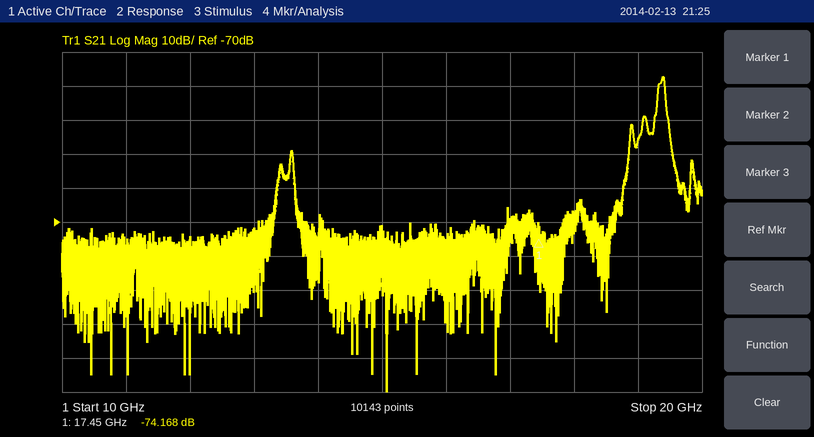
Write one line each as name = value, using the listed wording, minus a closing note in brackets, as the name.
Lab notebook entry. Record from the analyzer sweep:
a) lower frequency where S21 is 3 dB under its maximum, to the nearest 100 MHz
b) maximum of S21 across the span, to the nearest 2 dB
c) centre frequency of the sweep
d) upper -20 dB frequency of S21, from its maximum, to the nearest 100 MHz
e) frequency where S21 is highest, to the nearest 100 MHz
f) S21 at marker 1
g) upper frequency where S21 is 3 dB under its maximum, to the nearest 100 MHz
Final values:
lower frequency where S21 is 3 dB under its maximum, to the nearest 100 MHz = 19.3 GHz
maximum of S21 across the span, to the nearest 2 dB = -28 dB
centre frequency of the sweep = 15 GHz
upper -20 dB frequency of S21, from its maximum, to the nearest 100 MHz = 19.5 GHz
frequency where S21 is highest, to the nearest 100 MHz = 19.4 GHz
S21 at marker 1 = -74.168 dB
upper frequency where S21 is 3 dB under its maximum, to the nearest 100 MHz = 19.4 GHz
